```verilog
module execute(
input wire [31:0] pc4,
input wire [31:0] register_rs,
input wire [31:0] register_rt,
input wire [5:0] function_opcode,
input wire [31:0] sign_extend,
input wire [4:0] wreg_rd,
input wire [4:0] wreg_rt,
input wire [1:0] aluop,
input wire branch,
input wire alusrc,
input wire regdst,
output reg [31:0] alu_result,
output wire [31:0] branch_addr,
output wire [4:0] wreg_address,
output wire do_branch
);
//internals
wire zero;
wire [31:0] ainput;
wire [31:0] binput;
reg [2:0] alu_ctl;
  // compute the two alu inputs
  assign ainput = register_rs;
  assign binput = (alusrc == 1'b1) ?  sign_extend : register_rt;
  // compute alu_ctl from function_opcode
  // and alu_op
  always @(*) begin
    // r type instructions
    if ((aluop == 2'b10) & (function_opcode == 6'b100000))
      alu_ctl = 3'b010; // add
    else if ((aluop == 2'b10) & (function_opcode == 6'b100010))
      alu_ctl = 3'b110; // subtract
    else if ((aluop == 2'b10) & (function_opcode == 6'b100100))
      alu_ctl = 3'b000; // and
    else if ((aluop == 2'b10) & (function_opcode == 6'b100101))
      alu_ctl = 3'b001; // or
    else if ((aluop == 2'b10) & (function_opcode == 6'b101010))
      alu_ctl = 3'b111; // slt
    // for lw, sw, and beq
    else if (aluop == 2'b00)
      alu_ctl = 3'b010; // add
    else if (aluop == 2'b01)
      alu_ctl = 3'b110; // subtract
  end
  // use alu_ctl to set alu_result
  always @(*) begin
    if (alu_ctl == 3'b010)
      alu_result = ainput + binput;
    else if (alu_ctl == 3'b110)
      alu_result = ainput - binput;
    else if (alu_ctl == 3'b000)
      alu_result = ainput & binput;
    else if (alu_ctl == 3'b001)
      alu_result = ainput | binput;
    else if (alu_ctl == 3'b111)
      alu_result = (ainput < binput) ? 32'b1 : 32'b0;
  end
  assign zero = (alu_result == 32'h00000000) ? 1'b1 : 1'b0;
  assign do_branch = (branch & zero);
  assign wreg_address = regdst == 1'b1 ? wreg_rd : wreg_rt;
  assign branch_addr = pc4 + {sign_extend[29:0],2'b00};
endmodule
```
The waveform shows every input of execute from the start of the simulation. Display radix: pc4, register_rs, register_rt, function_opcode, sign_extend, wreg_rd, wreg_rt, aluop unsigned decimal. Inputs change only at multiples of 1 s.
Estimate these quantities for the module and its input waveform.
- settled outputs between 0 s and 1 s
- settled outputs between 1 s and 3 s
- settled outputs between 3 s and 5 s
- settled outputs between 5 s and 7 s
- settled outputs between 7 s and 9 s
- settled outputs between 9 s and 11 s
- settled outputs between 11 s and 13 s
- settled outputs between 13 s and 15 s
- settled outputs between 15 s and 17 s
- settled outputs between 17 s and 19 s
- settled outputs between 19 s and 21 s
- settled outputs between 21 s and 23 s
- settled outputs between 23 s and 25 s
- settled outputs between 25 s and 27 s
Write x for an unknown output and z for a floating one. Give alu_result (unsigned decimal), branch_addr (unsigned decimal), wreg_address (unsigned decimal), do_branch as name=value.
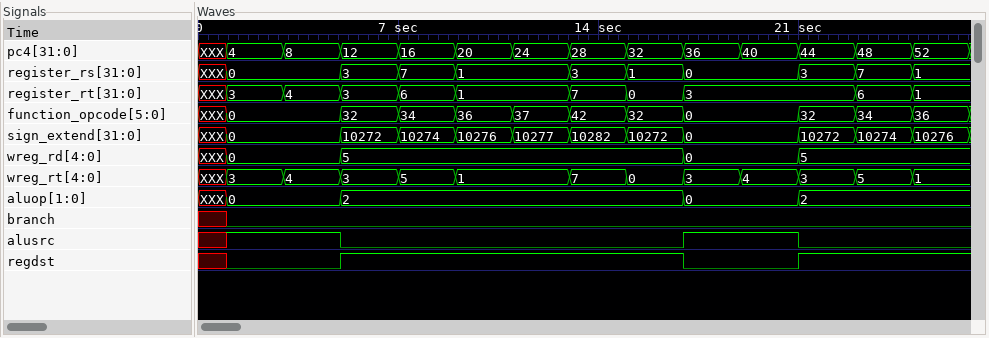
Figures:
alu_result=x, branch_addr=x, wreg_address=x, do_branch=x
alu_result=0, branch_addr=4, wreg_address=3, do_branch=0
alu_result=0, branch_addr=8, wreg_address=4, do_branch=0
alu_result=6, branch_addr=41100, wreg_address=5, do_branch=0
alu_result=1, branch_addr=41112, wreg_address=5, do_branch=0
alu_result=1, branch_addr=41124, wreg_address=5, do_branch=0
alu_result=1, branch_addr=41132, wreg_address=5, do_branch=0
alu_result=1, branch_addr=41156, wreg_address=5, do_branch=0
alu_result=1, branch_addr=41120, wreg_address=5, do_branch=0
alu_result=0, branch_addr=36, wreg_address=3, do_branch=0
alu_result=0, branch_addr=40, wreg_address=4, do_branch=0
alu_result=6, branch_addr=41132, wreg_address=5, do_branch=0
alu_result=1, branch_addr=41144, wreg_address=5, do_branch=0
alu_result=1, branch_addr=41156, wreg_address=5, do_branch=0
